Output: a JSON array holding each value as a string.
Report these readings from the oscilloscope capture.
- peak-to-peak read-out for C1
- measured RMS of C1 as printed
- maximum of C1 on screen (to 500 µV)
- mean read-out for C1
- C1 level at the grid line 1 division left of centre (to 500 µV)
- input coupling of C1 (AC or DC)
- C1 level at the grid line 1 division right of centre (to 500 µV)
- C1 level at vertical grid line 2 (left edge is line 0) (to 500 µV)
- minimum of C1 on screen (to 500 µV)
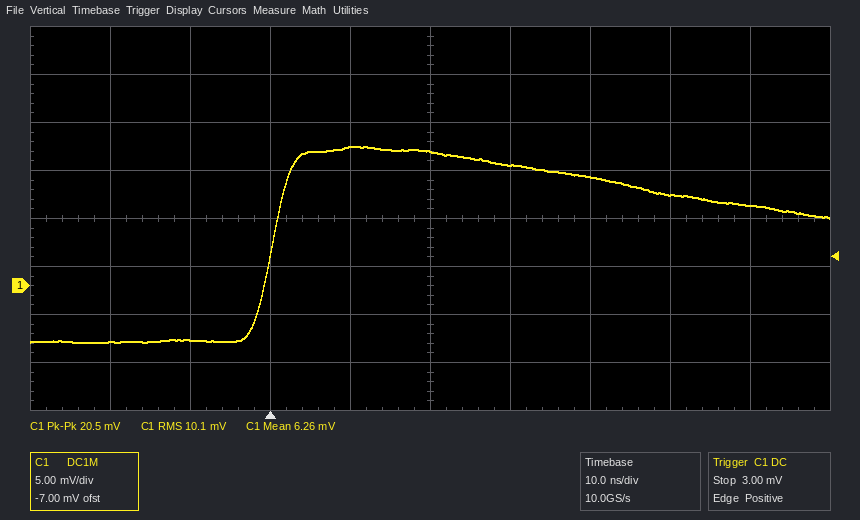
["20.5 mV", "10.1 mV", "14.5 mV", "6.26 mV", "14.5 mV", "DC", "12.5 mV", "-5.5 mV", "-6.0 mV"]
